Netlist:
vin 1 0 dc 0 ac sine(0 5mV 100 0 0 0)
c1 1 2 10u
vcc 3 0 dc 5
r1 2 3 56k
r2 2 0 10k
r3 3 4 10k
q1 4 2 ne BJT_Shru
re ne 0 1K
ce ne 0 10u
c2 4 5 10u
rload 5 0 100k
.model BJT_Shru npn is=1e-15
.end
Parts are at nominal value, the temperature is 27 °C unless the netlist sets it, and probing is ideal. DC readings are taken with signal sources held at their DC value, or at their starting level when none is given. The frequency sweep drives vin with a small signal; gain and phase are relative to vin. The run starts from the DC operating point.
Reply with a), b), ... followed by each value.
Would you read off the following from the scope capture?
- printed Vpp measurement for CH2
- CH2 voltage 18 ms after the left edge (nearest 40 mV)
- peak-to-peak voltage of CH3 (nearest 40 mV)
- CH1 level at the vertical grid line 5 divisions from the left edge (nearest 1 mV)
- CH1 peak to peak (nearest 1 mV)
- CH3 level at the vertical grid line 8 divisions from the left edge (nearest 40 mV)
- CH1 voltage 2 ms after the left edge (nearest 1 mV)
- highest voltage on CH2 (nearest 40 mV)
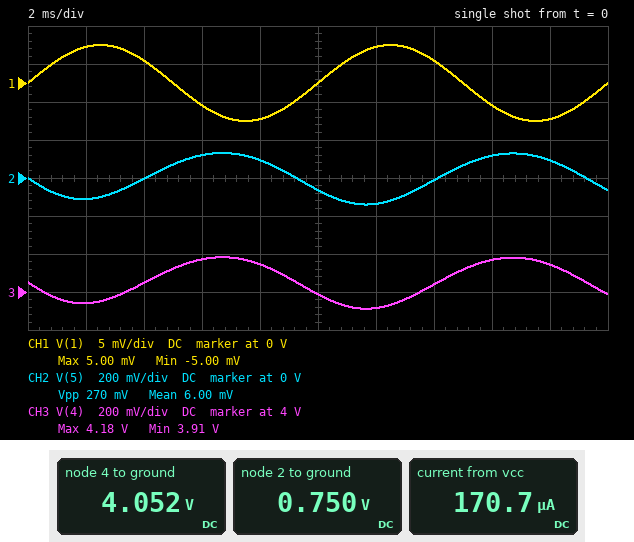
a) 270 mV
b) 80 mV
c) 280 mV
d) 0 V
e) 10 mV
f) 4.16 V
g) 5 mV
h) 120 mV
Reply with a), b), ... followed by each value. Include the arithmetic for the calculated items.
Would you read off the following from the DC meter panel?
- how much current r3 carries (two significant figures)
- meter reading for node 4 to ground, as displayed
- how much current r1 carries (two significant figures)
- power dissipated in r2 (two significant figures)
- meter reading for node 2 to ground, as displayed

a) (5 V - 4.052 V) / 10 kΩ = 95 µA
b) 4.052 V
c) (5 V - 750 mV) / 56 kΩ = 76 µA
d) (750 mV)^2 / 10 kΩ = 56 µW
e) 0.750 V
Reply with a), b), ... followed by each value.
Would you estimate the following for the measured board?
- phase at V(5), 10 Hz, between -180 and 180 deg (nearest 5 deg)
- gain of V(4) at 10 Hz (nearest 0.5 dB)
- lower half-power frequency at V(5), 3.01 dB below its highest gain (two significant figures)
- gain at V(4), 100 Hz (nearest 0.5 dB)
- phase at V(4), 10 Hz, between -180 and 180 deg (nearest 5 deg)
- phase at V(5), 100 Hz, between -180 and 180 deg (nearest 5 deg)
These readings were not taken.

a) -145 deg
b) 18.0 dB
c) 72 Hz
d) 28.5 dB
e) -145 deg
f) -150 deg
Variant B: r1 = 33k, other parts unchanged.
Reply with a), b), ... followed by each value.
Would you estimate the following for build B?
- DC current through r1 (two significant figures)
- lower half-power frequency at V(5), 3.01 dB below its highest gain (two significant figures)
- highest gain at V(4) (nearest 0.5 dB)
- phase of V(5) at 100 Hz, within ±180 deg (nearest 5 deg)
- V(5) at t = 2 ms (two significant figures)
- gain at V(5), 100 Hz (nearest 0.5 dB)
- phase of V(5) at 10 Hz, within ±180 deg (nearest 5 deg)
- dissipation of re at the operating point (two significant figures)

a) 120 µA
b) 290 Hz
c) 43.5 dB
d) -115 deg
e) -110 mV
f) 34.0 dB
g) -135 deg
h) 190 µW
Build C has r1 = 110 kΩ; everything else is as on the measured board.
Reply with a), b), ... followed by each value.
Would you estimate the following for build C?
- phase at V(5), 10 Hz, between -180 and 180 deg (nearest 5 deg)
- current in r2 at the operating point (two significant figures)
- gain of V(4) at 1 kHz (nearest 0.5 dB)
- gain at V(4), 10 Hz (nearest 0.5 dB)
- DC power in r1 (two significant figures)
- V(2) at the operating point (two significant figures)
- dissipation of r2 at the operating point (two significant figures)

a) -170 deg
b) 42 µA
c) -49.0 dB
d) -49.5 dB
e) 190 µW
f) 420 mV
g) 17 µW
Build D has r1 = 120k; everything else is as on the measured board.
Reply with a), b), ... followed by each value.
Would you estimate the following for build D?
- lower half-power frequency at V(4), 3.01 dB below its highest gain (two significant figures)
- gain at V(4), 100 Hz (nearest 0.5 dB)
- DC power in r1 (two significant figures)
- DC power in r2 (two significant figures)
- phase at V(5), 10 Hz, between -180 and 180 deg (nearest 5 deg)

a) 1.7 Hz
b) -60.0 dB
c) 180 µW
d) 15 µW
e) -170 deg
